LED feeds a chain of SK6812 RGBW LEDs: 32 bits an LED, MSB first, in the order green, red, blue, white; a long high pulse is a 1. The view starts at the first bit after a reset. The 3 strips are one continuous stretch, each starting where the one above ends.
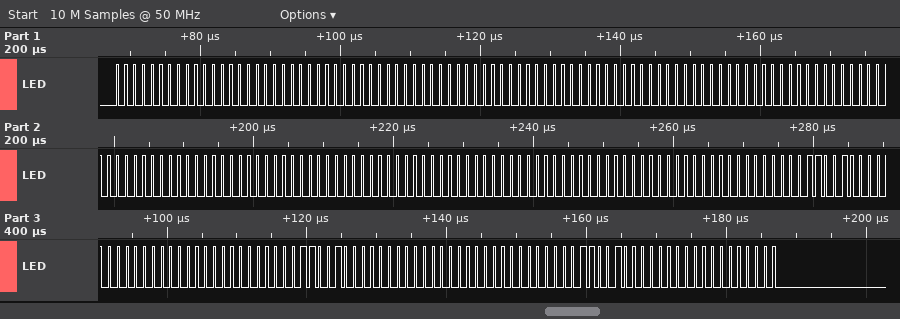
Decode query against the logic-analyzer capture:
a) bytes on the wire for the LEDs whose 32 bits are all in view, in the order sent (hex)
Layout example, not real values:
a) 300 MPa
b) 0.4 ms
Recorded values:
a) 00 00 00 00 00 00 00 00 00 00 00 00 00 00 00 00 00 00 00 00 00 64 00 00 00 64 00 00 00 64 00 00
